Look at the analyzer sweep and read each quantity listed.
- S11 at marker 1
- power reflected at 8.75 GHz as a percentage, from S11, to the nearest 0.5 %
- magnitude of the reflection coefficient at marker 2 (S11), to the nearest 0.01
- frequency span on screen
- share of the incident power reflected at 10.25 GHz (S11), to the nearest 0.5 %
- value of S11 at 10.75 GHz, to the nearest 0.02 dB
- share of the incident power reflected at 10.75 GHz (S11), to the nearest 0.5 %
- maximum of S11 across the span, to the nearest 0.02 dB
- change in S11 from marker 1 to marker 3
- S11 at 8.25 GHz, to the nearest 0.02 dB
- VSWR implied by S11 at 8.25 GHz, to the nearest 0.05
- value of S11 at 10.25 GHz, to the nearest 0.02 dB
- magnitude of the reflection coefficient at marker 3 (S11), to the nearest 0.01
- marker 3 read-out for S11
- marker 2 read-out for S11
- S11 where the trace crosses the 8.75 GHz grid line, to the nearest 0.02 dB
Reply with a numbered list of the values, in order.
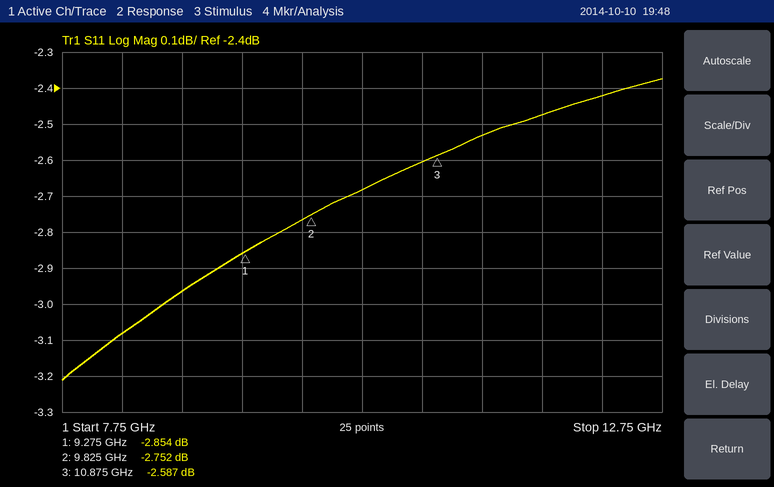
1. -2.854 dB
2. 50.5 %
3. 0.73
4. 5 GHz
5. 54.0 %
6. -2.60 dB
7. 55.0 %
8. -2.38 dB
9. 0.267 dB
10. -3.08 dB
11. 5.70
12. -2.68 dB
13. 0.74
14. -2.587 dB
15. -2.752 dB
16. -2.96 dB
